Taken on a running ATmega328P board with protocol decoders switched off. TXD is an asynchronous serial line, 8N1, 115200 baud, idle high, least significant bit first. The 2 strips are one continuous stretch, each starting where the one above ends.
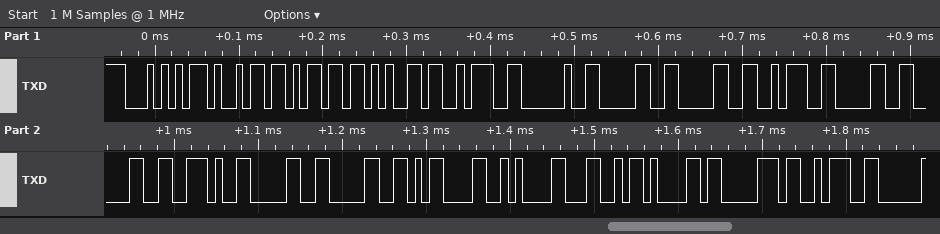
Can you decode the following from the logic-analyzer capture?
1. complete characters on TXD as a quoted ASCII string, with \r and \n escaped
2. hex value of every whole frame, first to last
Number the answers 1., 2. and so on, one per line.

1. "Time: 00:00.00\r\nLap:"
2. 54 69 6D 65 3A 20 30 30 3A 30 30 2E 30 30 0D 0A 4C 61 70 3A
